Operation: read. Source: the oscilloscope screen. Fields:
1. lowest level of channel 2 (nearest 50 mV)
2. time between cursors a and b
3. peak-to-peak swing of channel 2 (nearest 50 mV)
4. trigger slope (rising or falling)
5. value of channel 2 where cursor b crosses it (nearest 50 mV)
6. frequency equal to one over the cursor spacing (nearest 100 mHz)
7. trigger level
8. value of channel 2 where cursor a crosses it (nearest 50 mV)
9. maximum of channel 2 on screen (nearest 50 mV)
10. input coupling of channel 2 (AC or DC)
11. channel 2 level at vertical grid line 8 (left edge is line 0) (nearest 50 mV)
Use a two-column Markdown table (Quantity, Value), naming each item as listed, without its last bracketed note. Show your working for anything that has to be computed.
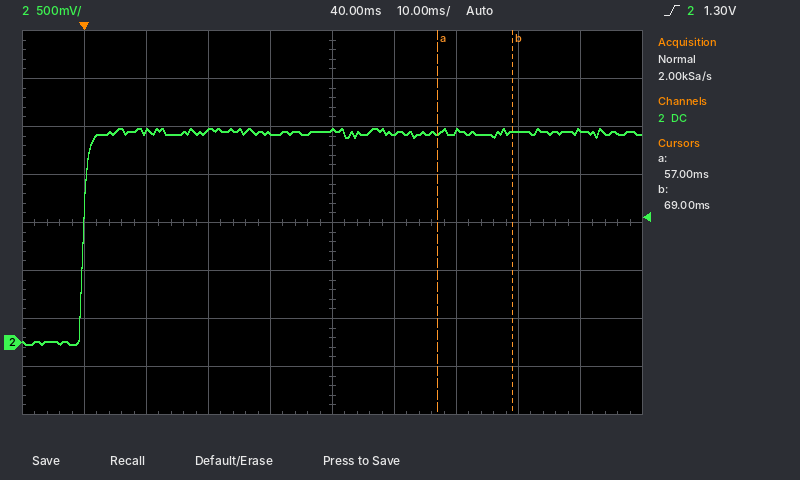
| Quantity | Value |
|---|---|
| lowest level of channel 2 | 0 mV |
| time between cursors a and b | 69 ms − (57 ms) = 12 ms |
| peak-to-peak swing of channel 2 | 2.25 V − (0 mV) = 2.25 V |
| trigger slope | rising |
| value of channel 2 where cursor b crosses it | 2.20 V |
| frequency equal to one over the cursor spacing | 1 / 12 ms ≈ 83.3 Hz |
| trigger level | 1.30 V |
| value of channel 2 where cursor a crosses it | 2.20 V |
| maximum of channel 2 on screen | 2.25 V |
| input coupling of channel 2 | DC |
| channel 2 level at vertical grid line 8 (left edge is line 0) | 2.20 V |
